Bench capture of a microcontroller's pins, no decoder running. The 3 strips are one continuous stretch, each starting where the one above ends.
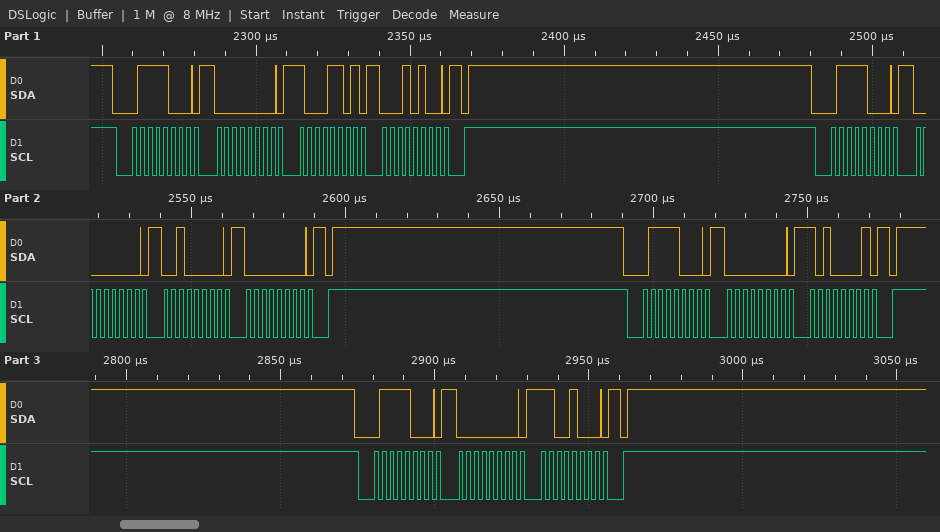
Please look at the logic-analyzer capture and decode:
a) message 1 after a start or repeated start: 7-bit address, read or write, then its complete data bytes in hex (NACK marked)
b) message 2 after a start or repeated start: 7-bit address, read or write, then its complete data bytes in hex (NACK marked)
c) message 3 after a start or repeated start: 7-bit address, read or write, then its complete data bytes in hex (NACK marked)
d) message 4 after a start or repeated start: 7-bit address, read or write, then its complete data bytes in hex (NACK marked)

0x3C write: 00 8D 14
0x3C write: 00 20 00
0x3C write: 00 A1
0x3C write: 00 C8
